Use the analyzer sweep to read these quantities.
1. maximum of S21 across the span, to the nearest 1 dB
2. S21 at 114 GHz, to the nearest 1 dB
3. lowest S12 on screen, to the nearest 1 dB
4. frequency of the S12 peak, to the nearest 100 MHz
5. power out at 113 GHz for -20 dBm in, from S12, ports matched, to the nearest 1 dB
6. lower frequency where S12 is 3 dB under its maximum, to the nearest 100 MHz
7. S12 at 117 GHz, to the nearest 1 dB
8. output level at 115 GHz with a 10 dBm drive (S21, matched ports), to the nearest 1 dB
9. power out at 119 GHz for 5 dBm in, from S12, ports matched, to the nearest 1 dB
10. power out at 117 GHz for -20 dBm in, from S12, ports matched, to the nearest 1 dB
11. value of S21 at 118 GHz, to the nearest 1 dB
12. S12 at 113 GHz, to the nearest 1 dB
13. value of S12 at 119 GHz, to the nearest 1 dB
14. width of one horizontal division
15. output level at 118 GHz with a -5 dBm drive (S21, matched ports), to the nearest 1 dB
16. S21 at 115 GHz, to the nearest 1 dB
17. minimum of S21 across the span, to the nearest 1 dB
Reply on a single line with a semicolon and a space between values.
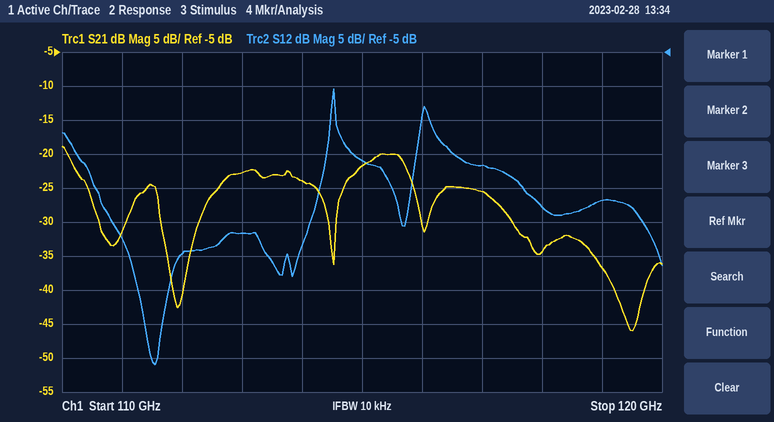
-19 dB; -24 dB; -51 dB; 114.5 GHz; -52 dBm; 114.5 GHz; -22 dB; -12 dBm; -22 dBm; -42 dBm; -34 dB; -32 dB; -27 dB; 1 GHz; -39 dBm; -22 dB; -46 dB
